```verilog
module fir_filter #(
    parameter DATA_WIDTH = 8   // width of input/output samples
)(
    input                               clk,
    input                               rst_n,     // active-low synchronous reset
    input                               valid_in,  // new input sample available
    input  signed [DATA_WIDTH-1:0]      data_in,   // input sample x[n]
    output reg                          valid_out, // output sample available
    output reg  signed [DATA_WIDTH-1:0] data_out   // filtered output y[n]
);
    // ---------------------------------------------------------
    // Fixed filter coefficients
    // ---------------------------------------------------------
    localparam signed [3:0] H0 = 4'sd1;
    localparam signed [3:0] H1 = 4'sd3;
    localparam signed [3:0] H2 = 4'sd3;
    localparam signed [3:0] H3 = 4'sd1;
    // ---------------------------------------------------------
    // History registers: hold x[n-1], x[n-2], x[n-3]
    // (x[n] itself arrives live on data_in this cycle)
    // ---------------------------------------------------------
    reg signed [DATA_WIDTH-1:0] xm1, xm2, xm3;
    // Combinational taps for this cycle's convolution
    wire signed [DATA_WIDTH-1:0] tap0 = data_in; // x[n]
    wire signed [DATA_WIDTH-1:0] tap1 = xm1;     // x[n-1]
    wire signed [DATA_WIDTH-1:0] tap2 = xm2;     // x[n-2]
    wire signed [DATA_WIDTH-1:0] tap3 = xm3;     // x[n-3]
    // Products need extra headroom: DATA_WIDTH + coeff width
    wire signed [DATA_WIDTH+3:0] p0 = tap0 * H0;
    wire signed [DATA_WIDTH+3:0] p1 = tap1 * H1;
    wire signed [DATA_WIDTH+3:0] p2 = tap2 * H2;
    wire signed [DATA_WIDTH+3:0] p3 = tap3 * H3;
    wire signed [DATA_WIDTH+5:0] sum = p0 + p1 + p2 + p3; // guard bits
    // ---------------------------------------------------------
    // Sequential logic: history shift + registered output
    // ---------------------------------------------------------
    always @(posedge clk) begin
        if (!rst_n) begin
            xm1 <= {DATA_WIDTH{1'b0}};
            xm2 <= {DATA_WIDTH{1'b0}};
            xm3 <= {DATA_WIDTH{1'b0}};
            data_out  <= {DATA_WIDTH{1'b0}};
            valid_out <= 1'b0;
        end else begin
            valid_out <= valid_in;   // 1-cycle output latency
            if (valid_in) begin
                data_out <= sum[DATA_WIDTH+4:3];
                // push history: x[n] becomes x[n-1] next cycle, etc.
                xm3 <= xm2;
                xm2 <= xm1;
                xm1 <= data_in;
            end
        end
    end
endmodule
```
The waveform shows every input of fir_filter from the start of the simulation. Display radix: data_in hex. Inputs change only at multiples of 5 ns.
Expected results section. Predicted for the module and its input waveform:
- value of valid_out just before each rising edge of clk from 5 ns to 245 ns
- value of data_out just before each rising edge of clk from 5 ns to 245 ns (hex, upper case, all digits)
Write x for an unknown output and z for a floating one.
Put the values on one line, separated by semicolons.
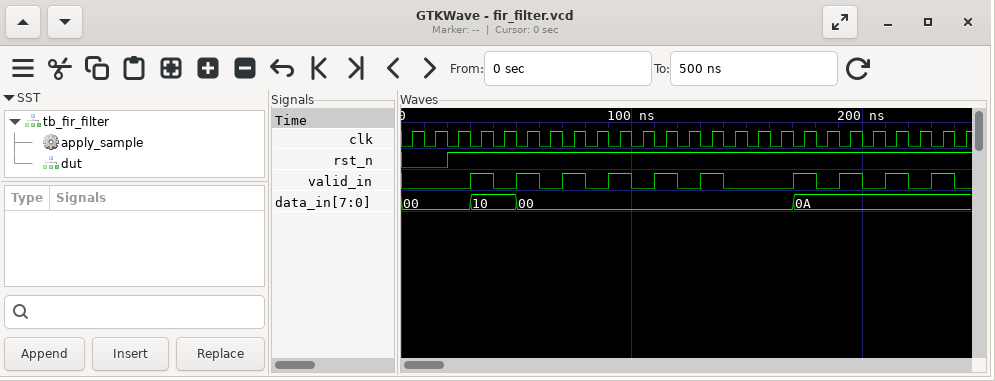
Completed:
x 0 0 0 1 0 1 0 1 0 1 0 1 0 1 0 0 0 1 0 1 0 1 0 1; x, 00, 00, 00, 02, 02, 06, 06, 06, 06, 02, 02, 00, 00, 00, 00, 00, 00, 01, 01, 05, 05, 08, 08, 0A
